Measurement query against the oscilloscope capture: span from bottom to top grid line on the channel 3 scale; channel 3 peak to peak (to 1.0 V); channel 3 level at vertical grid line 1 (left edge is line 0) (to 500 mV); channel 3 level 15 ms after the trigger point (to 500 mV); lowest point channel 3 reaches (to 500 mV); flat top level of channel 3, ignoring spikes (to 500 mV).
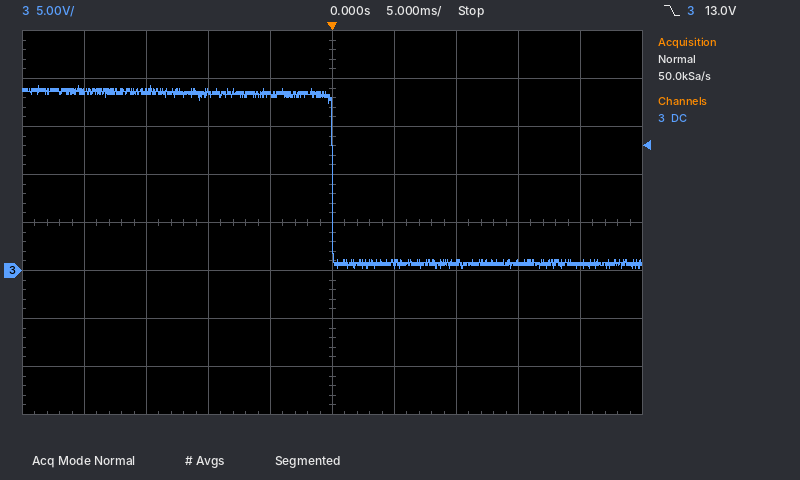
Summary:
40 V
19.0 V
18.5 V
1.0 V
0.0 V
18.5 V
